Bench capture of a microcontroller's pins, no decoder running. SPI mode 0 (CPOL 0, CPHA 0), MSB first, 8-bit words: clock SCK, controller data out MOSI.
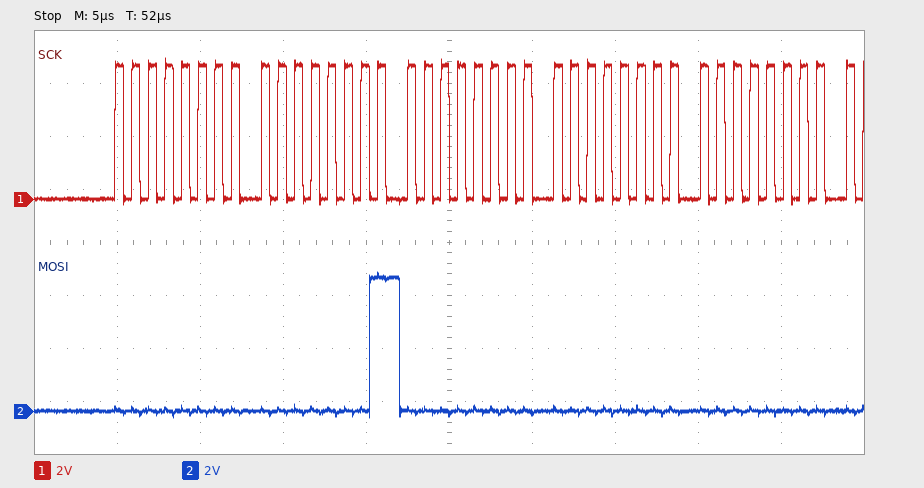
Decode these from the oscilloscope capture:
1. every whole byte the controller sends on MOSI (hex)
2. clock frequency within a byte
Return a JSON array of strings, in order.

["00 01 00 00 00", "1 MHz"]
